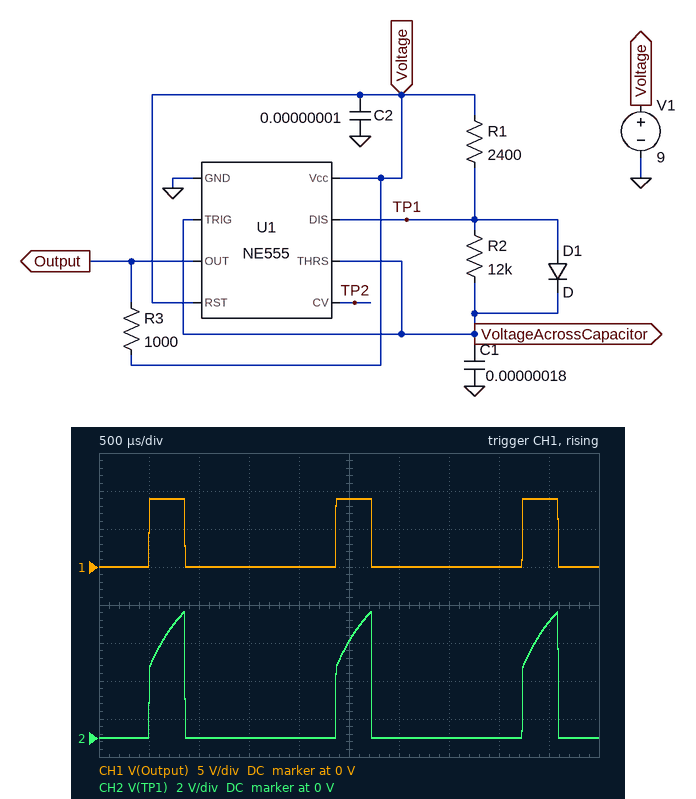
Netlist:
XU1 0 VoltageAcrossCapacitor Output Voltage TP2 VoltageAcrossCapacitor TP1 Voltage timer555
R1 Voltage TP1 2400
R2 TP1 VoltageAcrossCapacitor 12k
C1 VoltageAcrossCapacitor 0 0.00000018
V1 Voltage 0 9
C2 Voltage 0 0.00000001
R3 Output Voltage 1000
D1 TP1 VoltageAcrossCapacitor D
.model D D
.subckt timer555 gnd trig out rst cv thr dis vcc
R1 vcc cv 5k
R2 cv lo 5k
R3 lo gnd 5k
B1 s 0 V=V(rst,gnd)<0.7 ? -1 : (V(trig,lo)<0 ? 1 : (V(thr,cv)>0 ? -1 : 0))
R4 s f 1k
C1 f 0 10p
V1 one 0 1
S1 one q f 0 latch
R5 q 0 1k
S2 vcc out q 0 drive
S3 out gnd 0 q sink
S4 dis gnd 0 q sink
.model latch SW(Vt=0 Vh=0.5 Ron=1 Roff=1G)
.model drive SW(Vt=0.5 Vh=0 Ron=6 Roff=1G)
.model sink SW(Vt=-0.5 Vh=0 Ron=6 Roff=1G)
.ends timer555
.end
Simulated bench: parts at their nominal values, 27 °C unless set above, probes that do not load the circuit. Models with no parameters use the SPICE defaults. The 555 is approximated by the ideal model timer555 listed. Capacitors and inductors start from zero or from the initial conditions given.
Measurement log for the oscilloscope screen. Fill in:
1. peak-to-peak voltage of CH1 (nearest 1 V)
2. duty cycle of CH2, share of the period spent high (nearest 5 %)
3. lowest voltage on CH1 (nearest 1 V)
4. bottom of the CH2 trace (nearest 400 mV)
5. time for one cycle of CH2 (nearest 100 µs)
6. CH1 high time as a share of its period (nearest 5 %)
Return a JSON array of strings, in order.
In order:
["9 V", "20 %", "0 V", "0 V", "1.9 ms", "20 %"]
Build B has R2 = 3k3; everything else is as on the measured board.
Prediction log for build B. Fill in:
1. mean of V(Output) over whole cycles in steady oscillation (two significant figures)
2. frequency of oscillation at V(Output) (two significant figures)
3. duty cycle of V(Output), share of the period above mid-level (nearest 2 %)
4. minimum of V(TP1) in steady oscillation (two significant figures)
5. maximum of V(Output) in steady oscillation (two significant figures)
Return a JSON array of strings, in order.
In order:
["4.2 V", "1.3 kHz", "46 %", "28 mV", "9.0 V"]
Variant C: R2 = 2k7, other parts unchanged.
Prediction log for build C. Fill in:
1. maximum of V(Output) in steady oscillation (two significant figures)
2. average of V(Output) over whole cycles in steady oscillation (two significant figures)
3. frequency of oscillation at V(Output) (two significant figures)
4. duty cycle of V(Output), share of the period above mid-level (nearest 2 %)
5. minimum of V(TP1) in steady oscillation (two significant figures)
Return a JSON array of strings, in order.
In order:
["9.0 V", "4.6 V", "1.4 kHz", "52 %", "29 mV"]
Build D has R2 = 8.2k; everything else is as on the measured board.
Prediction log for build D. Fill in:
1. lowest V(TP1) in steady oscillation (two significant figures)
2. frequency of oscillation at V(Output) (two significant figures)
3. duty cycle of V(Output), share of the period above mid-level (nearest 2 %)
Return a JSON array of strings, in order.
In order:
["25 mV", "720 Hz", "26 %"]
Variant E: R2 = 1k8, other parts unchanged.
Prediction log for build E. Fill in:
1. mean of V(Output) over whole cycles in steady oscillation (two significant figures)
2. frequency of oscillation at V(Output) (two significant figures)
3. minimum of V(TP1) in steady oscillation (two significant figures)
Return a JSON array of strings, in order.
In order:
["5.5 V", "1.7 kHz", "32 mV"]
